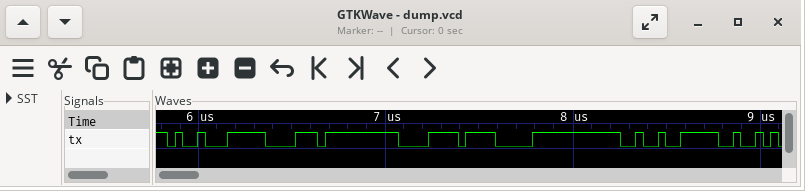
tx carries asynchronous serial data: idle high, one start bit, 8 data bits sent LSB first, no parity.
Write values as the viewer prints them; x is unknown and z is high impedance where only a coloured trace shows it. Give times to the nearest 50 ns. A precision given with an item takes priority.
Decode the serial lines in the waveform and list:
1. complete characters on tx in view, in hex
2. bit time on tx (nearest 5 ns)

89, B8, 78, F0, 92
40 ns
